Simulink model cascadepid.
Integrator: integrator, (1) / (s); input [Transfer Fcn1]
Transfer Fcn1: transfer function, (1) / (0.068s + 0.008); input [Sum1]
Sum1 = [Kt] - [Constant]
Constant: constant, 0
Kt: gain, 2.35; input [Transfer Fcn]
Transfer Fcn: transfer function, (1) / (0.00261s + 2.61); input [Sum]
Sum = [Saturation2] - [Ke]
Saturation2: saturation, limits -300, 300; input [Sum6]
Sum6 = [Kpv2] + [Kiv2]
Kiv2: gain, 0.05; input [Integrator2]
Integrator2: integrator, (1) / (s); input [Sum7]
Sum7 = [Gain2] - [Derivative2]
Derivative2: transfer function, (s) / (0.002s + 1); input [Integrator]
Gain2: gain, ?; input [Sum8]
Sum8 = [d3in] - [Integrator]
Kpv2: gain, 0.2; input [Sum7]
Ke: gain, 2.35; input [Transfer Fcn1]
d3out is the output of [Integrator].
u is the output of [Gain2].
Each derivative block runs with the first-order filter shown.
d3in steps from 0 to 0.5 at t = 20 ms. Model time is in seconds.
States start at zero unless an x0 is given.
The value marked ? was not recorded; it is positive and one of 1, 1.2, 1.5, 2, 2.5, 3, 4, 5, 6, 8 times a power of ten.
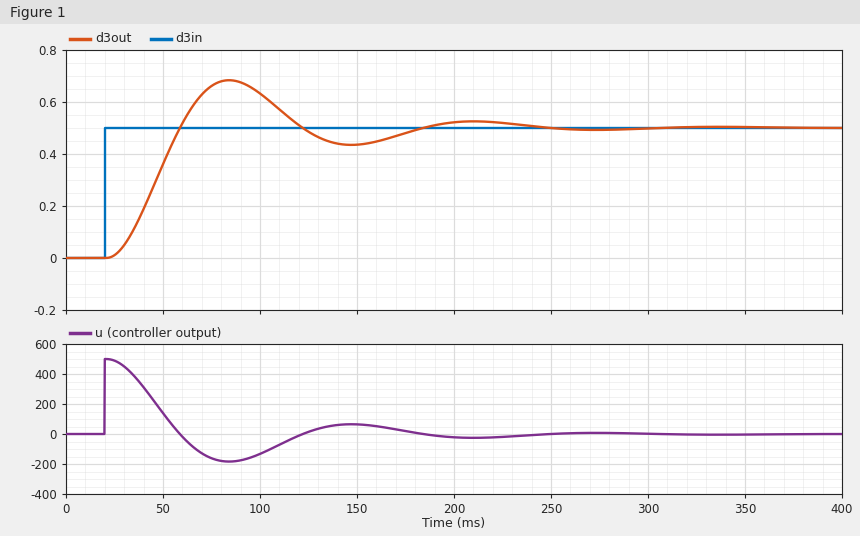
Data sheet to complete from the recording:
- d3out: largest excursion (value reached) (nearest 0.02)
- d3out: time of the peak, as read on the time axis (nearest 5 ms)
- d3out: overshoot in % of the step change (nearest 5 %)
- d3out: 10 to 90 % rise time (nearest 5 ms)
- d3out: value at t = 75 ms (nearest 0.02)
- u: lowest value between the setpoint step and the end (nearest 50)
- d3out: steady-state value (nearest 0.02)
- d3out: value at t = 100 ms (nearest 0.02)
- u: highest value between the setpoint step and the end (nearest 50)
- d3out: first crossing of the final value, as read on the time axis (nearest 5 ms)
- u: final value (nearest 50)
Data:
0.68
85 ms
35 %
25 ms
0.66
-200
0.50
0.64
500
60 ms
0
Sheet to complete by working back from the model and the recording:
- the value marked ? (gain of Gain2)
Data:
1000
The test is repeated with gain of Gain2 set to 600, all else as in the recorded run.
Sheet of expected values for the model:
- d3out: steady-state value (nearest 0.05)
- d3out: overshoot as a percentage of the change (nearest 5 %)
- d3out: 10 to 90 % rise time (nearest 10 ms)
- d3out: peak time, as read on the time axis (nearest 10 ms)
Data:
0.50
25 %
40 ms
110 ms
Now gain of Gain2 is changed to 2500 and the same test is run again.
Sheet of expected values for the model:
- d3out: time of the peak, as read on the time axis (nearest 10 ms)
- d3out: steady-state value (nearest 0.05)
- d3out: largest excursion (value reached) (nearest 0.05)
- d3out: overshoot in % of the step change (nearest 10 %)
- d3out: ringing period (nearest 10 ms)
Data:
60 ms
0.50
0.80
60 %
80 ms
